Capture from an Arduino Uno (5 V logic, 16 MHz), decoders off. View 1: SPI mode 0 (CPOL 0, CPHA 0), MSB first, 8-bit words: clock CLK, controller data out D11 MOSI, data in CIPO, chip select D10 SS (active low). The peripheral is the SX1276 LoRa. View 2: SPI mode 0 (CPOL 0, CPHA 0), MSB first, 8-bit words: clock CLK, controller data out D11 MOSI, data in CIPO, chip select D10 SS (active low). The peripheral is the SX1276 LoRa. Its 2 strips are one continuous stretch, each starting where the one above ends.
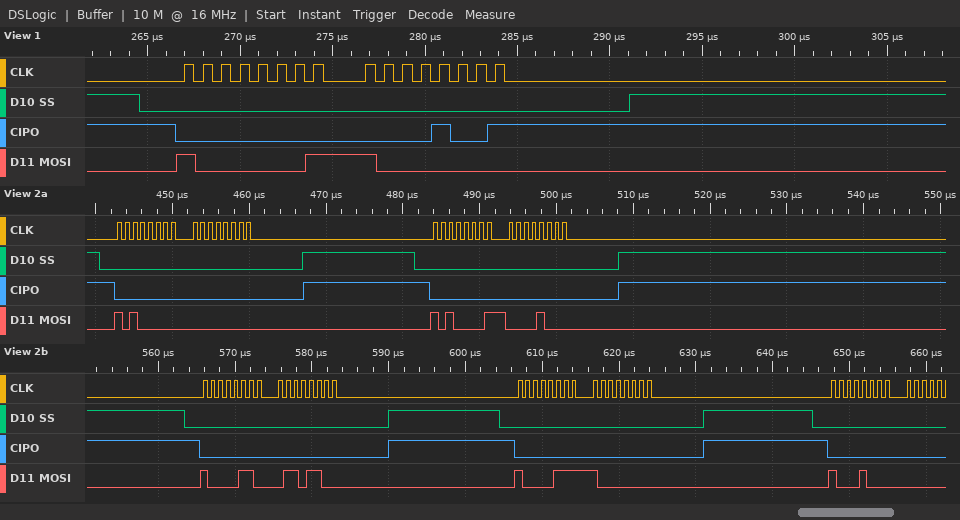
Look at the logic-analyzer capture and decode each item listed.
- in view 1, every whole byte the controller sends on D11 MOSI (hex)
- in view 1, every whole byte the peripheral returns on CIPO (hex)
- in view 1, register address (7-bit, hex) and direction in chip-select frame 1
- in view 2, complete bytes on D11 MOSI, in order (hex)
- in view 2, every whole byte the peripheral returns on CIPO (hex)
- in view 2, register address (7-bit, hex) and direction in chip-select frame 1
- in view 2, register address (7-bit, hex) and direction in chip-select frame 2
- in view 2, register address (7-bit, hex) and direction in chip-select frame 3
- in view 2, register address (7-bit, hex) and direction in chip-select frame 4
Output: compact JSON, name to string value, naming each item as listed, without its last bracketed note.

{"in view 1, every whole byte the controller sends on D11 MOSI": "0x81 0x80", "in view 1, every whole byte the peripheral returns on CIPO": "0x00 0x09", "in view 1, register address (7-bit, hex) and direction in chip-select frame 1": "0x01 write", "in view 2, complete bytes on D11 MOSI, in order": "0xA0 0x00 0xA1 0x08 0x86 0x6C 0x87 0x80 0x88", "in view 2, every whole byte the peripheral returns on CIPO": "0x00 0x00 0x00 0x00 0x00 0x00 0x00 0x00 0x00", "in view 2, register address (7-bit, hex) and direction in chip-select frame 1": "0x20 write", "in view 2, register address (7-bit, hex) and direction in chip-select frame 2": "0x21 write", "in view 2, register address (7-bit, hex) and direction in chip-select frame 3": "0x06 write", "in view 2, register address (7-bit, hex) and direction in chip-select frame 4": "0x07 write"}
